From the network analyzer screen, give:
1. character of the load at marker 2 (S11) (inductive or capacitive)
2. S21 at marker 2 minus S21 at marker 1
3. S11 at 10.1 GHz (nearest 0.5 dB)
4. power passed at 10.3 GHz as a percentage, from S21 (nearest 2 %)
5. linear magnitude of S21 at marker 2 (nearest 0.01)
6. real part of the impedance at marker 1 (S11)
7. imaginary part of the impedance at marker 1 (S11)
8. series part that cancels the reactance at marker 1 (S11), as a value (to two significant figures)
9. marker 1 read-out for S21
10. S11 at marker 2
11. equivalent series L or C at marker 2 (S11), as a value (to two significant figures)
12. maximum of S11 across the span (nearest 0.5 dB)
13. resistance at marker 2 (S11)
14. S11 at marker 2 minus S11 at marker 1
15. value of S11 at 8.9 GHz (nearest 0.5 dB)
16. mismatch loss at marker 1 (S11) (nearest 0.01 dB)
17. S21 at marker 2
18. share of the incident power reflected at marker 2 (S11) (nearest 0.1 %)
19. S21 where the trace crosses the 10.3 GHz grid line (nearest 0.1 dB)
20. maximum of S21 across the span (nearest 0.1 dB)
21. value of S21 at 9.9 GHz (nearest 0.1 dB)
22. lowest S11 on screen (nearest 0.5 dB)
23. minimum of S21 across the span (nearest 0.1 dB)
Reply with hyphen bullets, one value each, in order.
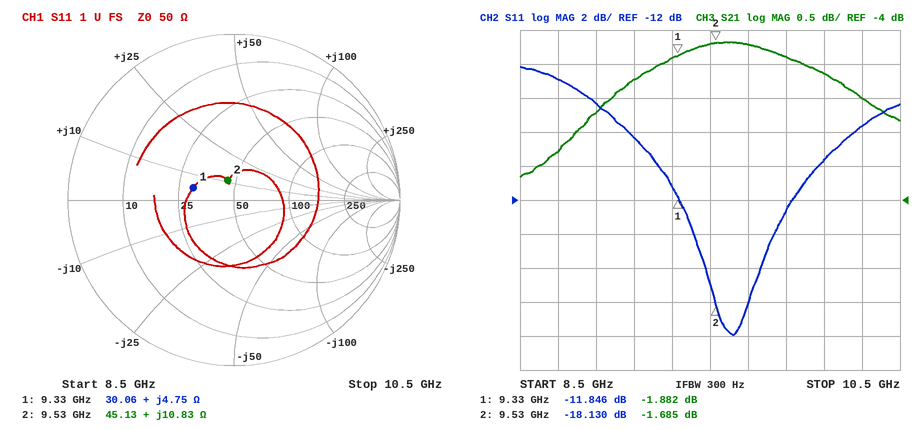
- inductive
- 0.197 dB
- -9.5 dB
- 56 %
- 0.82
- 30.06 Ω
- +4.75 Ω
- 3.6 pF
- -1.882 dB
- -18.130 dB
- 180 pH
- -4.0 dB
- 45.13 Ω
- -6.284 dB
- -6.5 dB
- 0.29 dB
- -1.685 dB
- 1.5 %
- -2.5 dB
- -1.7 dB
- -1.9 dB
- -20.0 dB
- -3.7 dB
